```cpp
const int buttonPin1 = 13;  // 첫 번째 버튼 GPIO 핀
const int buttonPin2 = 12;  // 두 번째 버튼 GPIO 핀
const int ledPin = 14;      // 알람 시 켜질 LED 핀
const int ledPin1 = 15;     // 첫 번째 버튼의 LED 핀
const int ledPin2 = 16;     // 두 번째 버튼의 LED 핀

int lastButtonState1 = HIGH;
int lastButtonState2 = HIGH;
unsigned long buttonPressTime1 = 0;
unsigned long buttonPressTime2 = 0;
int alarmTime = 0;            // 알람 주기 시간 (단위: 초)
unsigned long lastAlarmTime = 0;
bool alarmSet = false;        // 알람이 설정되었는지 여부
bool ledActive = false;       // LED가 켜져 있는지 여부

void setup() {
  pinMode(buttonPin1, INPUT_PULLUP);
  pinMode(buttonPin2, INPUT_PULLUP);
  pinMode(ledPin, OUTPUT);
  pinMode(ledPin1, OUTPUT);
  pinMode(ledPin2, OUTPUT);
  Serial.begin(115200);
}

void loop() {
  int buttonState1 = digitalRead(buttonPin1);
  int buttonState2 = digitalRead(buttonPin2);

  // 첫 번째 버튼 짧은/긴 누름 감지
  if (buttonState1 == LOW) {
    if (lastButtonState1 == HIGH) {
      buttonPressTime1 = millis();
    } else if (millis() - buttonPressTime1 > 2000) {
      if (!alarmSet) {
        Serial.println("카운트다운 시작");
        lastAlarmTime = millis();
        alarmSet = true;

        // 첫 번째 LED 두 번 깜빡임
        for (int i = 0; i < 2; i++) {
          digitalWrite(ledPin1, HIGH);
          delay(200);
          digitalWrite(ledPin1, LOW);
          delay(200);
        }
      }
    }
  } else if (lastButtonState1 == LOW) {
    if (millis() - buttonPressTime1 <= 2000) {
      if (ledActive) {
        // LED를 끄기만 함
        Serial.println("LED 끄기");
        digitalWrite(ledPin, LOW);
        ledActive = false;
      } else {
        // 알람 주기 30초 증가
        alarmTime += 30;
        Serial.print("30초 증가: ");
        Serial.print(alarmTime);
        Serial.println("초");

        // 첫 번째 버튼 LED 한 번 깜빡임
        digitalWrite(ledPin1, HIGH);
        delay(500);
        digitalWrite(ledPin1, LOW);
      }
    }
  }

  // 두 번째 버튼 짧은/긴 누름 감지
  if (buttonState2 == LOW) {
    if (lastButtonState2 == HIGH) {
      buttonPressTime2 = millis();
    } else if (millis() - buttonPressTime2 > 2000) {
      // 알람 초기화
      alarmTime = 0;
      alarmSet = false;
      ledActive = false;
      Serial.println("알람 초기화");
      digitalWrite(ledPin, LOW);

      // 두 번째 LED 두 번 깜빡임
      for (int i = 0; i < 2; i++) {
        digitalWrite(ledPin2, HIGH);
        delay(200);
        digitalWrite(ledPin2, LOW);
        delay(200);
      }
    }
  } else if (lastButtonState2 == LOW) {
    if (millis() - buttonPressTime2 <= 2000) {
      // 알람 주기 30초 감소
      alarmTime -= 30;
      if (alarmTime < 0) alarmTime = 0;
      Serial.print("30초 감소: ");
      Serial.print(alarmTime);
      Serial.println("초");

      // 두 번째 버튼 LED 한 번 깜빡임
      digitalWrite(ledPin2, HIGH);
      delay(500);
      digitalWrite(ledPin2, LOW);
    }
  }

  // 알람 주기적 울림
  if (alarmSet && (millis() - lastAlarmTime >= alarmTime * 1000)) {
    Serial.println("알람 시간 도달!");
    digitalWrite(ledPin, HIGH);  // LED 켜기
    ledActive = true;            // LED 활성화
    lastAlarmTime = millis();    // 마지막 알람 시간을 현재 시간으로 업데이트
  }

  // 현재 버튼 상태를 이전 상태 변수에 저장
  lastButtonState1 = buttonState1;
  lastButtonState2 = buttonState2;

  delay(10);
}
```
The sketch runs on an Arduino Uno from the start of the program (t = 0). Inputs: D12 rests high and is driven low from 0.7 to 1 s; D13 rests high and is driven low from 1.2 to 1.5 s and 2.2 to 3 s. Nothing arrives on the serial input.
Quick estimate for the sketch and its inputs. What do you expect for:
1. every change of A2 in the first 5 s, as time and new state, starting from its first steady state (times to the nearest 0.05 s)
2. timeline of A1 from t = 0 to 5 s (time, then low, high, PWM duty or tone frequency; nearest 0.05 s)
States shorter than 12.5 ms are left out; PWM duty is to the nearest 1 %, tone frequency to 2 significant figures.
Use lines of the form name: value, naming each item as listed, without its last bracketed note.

every change of A2 in the first 5 s, as time and new state, starting from its first steady state: 0 s low; 1 s high; 1.5 s low
timeline of A1 from t = 0 to 5 s: 0 s low; 3 s high; 3.5 s low
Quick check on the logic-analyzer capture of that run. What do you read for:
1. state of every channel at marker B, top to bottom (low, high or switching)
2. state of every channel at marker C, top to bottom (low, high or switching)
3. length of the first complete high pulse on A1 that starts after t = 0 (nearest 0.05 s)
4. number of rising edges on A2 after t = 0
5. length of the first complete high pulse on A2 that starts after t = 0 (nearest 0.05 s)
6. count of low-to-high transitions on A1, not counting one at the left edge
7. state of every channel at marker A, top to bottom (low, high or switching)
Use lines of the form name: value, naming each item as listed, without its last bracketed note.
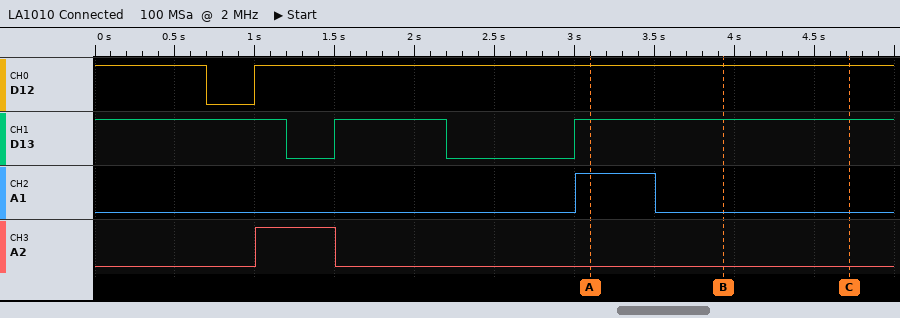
state of every channel at marker B, top to bottom: D12 high, D13 high, A1 low, A2 low
state of every channel at marker C, top to bottom: D12 high, D13 high, A1 low, A2 low
length of the first complete high pulse on A1 that starts after t = 0: 0.50 s
number of rising edges on A2 after t = 0: 1
length of the first complete high pulse on A2 that starts after t = 0: 0.50 s
count of low-to-high transitions on A1, not counting one at the left edge: 1
state of every channel at marker A, top to bottom: D12 high, D13 high, A1 high, A2 low
